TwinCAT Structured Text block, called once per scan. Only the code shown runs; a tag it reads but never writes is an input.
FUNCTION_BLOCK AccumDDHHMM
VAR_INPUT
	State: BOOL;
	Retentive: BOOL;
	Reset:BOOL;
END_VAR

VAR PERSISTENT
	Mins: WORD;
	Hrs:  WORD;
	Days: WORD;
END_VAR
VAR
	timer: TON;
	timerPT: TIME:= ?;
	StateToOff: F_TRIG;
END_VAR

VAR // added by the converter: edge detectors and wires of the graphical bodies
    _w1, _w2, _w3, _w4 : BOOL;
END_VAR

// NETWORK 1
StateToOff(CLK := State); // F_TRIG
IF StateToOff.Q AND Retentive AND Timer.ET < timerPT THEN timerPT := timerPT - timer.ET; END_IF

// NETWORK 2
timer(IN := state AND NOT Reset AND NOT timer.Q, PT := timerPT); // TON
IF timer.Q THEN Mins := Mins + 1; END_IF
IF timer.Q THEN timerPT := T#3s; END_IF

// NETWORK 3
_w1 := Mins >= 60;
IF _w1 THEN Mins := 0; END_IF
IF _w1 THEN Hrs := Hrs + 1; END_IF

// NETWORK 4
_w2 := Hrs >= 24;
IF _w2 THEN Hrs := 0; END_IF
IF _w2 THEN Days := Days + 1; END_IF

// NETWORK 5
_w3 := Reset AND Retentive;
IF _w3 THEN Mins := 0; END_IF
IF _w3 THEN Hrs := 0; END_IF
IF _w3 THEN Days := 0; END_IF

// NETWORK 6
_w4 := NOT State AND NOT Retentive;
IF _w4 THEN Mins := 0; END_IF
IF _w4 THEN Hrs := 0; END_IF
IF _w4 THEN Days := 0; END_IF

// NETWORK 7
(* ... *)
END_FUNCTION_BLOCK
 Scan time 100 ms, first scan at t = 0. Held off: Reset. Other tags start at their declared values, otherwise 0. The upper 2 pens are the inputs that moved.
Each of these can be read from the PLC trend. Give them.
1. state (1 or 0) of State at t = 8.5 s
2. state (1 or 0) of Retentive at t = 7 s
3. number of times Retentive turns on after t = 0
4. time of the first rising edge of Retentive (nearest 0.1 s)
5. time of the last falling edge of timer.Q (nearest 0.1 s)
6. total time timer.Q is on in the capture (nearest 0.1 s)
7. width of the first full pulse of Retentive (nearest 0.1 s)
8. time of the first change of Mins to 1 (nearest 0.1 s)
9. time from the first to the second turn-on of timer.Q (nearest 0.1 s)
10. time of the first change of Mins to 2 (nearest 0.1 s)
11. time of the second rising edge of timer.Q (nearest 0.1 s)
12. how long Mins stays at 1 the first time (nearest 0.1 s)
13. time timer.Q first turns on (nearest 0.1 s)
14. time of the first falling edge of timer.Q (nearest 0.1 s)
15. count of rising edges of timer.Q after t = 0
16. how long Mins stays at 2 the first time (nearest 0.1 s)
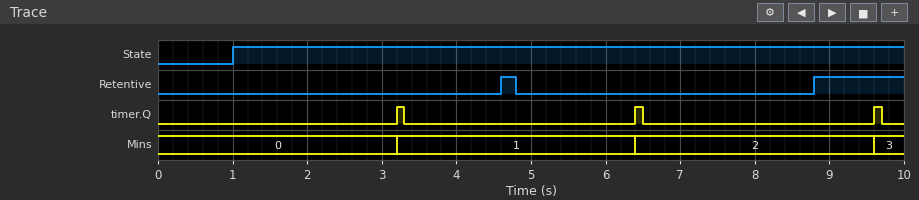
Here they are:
1
0
2
4.6 s
9.7 s
0.3 s
0.2 s
3.2 s
3.2 s
6.4 s
6.4 s
3.2 s
3.2 s
3.3 s
3
3.2 s
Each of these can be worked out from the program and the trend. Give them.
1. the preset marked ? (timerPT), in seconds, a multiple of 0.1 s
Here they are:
2.2 s
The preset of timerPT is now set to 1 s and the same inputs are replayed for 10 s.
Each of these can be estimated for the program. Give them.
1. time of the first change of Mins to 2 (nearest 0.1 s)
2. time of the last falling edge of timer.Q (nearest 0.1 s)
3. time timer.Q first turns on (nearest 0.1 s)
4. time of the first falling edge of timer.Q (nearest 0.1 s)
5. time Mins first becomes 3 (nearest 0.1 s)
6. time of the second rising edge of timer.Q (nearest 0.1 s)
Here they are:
5.2 s
8.5 s
2.0 s
2.1 s
8.4 s
5.2 s
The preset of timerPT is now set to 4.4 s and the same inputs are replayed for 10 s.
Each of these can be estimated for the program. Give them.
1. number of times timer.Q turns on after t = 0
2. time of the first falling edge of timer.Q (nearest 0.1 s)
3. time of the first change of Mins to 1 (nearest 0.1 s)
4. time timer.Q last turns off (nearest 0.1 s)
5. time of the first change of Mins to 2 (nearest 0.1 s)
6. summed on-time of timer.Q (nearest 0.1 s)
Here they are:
2
5.5 s
5.4 s
8.7 s
8.6 s
0.2 s
